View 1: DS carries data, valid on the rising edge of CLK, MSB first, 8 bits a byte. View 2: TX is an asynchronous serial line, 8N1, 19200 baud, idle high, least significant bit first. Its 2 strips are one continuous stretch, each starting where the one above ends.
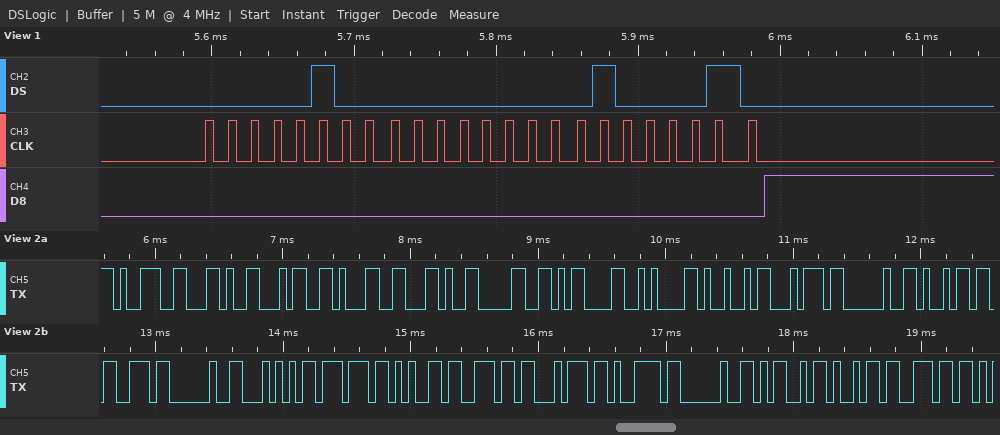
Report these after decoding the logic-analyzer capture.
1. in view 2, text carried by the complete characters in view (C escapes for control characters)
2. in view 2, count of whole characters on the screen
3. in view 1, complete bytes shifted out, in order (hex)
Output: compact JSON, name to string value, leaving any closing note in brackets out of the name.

{"in view 2, text carried by the complete characters in view": "\"9,41,0\\r\\nIt is Twenty Min\"", "in view 2, count of whole characters on the screen": "24", "in view 1, complete bytes shifted out, in order": "04 00 42"}
